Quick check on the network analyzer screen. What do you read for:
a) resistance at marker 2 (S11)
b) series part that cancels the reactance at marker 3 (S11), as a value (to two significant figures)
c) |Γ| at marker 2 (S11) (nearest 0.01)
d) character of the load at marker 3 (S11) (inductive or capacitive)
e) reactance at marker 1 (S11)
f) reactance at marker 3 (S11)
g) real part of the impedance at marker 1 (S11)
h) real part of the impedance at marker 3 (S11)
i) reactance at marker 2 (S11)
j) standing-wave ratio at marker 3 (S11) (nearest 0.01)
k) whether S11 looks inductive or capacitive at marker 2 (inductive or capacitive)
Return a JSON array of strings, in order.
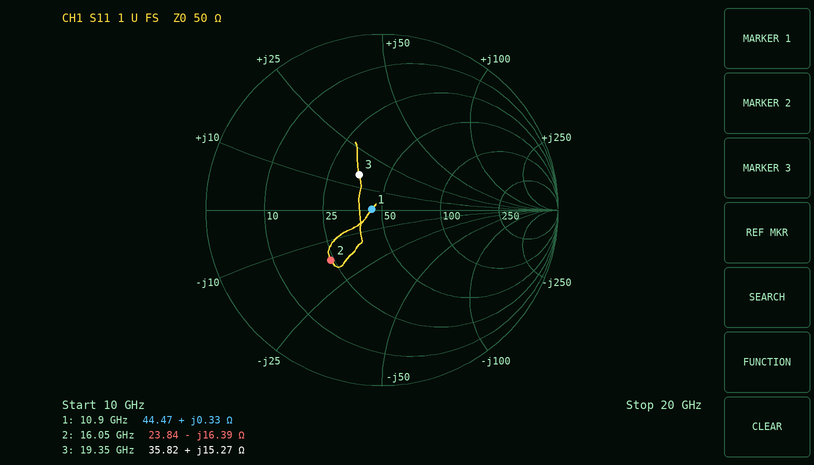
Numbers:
["23.84 Ω", "540 fF", "0.41", "inductive", "+0.33 Ω", "+15.27 Ω", "44.47 Ω", "35.82 Ω", "-16.39 Ω", "1.63", "capacitive"]
